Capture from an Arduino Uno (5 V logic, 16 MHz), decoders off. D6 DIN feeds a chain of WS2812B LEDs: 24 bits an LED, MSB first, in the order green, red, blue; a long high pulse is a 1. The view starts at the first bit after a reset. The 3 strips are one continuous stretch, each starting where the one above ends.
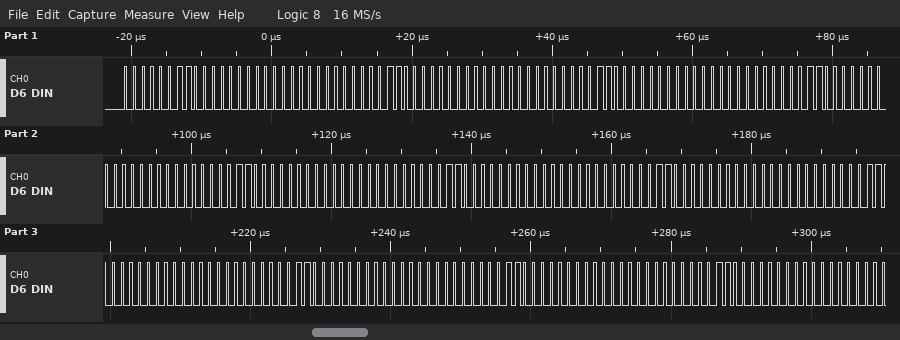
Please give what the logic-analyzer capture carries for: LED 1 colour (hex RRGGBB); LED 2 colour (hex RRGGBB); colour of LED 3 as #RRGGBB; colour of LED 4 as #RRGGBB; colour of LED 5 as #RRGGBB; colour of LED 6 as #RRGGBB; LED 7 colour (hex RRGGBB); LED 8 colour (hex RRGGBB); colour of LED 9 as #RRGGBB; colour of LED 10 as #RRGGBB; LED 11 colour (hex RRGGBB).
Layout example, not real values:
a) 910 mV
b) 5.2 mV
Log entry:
a) #000300
b) #000300
c) #000300
d) #000300
e) #000300
f) #000300
g) #000300
h) #000300
i) #000300
j) #000300
k) #000300
